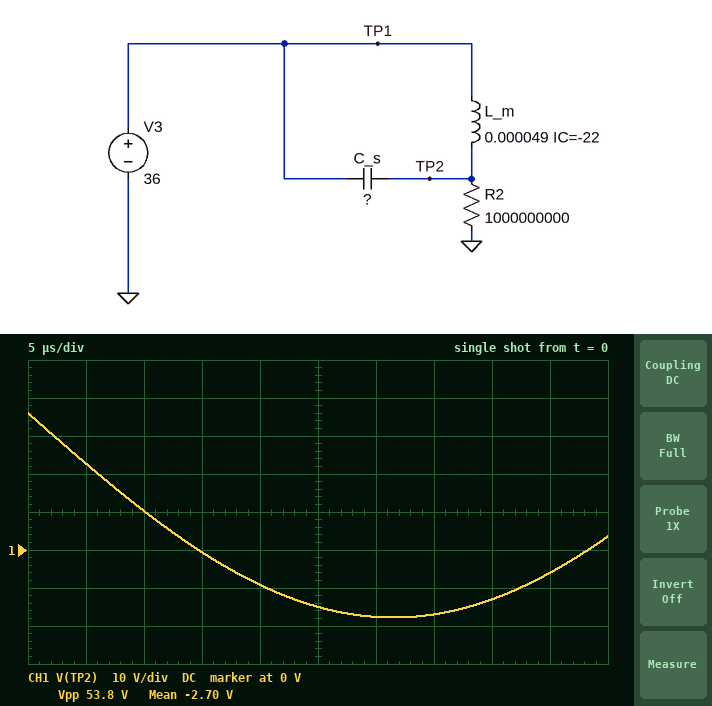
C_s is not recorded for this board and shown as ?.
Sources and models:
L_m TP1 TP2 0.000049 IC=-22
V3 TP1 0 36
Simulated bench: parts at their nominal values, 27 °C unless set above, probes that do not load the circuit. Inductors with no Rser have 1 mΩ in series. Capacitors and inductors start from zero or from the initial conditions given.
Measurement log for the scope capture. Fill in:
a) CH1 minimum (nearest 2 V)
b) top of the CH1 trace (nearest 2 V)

-18 V
36 V
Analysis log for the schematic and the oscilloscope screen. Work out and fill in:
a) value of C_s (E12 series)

8.2 µF
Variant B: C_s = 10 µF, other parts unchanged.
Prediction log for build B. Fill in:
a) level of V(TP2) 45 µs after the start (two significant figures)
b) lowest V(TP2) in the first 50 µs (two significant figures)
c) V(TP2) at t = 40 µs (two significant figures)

-7.6 V
-13 V
-11 V
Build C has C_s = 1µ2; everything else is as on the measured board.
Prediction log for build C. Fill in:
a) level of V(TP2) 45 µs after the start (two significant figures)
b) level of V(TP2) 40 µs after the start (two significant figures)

93 V
160 V
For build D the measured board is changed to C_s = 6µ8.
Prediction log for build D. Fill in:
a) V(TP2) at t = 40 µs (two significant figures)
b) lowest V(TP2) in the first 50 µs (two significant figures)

-12 V
-23 V
